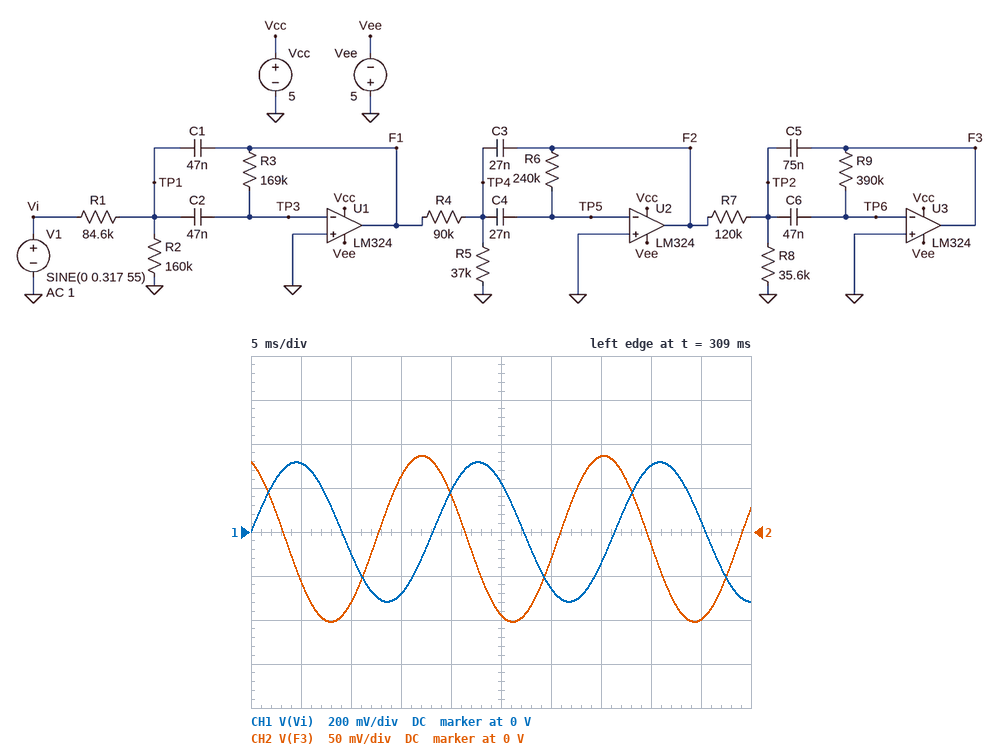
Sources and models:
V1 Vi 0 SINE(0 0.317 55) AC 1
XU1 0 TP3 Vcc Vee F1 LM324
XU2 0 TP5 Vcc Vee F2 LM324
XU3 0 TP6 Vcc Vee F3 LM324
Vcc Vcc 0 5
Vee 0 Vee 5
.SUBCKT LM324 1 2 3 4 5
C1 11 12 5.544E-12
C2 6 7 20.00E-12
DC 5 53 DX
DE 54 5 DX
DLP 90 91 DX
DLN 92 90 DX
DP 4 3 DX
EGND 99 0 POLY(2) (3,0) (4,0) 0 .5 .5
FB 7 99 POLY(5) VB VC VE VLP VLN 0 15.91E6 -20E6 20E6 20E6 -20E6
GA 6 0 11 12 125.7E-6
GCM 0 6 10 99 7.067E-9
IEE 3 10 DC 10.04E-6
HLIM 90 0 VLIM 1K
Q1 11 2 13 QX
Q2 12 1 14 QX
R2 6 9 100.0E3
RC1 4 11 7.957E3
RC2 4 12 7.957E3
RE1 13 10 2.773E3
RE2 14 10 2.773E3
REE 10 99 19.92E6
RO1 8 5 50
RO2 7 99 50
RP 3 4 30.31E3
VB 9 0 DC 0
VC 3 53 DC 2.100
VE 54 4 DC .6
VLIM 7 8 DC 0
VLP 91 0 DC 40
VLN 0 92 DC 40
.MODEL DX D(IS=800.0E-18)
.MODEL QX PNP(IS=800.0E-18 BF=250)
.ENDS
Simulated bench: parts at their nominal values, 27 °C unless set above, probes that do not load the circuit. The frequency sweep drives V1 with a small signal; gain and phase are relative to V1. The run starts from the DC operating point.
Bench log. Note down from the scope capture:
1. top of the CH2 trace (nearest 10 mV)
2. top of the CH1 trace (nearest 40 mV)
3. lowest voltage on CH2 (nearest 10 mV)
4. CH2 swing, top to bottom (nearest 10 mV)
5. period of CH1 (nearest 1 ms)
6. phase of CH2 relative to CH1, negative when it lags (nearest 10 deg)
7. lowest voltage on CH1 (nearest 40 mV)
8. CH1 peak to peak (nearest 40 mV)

90 mV
320 mV
-100 mV
190 mV
18 ms
110 deg
-320 mV
640 mV
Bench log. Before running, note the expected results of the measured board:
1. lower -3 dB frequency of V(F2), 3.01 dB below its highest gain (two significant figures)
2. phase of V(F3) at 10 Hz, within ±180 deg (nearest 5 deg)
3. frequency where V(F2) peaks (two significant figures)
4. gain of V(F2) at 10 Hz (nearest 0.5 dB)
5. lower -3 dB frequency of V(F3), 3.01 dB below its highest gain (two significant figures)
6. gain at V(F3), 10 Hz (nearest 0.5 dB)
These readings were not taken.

39 Hz
50 deg
65 Hz
-28.0 dB
24 Hz
-38.5 dB
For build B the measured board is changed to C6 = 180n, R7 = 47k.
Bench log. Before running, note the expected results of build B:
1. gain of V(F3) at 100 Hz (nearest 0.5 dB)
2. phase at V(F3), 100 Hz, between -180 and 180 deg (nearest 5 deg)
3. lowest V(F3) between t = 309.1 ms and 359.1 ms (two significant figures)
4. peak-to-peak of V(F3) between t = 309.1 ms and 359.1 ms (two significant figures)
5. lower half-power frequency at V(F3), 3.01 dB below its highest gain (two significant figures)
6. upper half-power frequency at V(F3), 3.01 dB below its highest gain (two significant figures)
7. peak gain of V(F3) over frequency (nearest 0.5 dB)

-14.5 dB
-15 deg
-220 mV
420 mV
15 Hz
70 Hz
-2.5 dB
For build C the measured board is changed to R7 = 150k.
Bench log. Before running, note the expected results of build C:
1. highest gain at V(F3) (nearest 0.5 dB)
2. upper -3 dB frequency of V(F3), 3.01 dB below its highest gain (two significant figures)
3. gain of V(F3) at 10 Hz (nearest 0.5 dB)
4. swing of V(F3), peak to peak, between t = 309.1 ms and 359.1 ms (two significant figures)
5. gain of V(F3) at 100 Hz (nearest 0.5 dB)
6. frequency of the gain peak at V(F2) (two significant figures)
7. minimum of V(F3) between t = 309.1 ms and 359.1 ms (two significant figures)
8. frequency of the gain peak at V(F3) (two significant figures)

-9.5 dB
55 Hz
-40.0 dB
150 mV
-24.5 dB
65 Hz
-82 mV
30 Hz
